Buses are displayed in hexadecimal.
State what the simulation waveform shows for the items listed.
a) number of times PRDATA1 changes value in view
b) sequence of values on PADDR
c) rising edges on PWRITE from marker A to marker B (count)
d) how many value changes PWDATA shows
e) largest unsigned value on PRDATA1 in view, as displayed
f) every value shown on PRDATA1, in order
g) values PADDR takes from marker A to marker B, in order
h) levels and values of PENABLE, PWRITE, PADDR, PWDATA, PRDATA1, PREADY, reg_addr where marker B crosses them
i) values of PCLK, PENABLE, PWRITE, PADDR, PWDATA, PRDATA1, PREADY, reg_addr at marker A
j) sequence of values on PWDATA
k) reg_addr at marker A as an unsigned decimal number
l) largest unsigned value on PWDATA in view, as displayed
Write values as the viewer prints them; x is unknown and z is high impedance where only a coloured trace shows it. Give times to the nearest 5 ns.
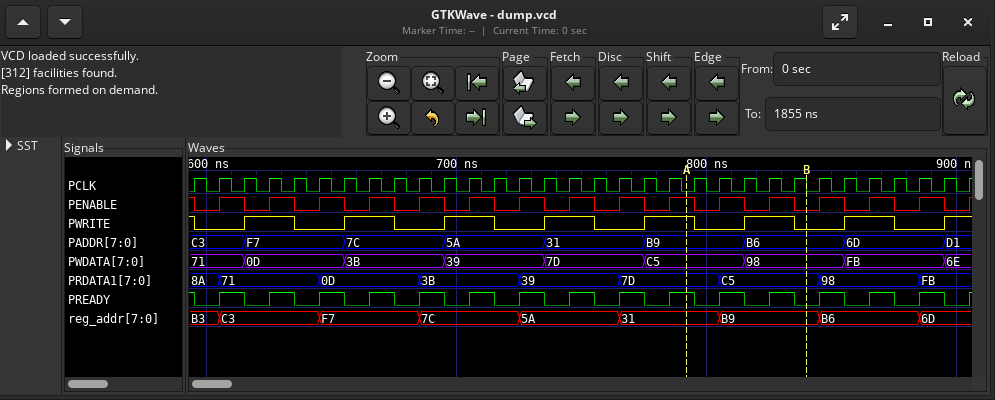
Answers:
8
C3, F7, 7C, 5A, 31, B9, B6, 6D, D1
1
8
FB
8A, 71, 0D, 3B, 39, 7D, C5, 98, FB
B9, B6
PENABLE=0, PWRITE=0, PADDR=B6, PWDATA=98, PRDATA1=C5, PREADY=0, reg_addr=B9
PCLK=0, PENABLE=1, PWRITE=1, PADDR=B9, PWDATA=C5, PRDATA1=7D, PREADY=1, reg_addr=31
71, 0D, 3B, 39, 7D, C5, 98, FB, 6E
49
FB
